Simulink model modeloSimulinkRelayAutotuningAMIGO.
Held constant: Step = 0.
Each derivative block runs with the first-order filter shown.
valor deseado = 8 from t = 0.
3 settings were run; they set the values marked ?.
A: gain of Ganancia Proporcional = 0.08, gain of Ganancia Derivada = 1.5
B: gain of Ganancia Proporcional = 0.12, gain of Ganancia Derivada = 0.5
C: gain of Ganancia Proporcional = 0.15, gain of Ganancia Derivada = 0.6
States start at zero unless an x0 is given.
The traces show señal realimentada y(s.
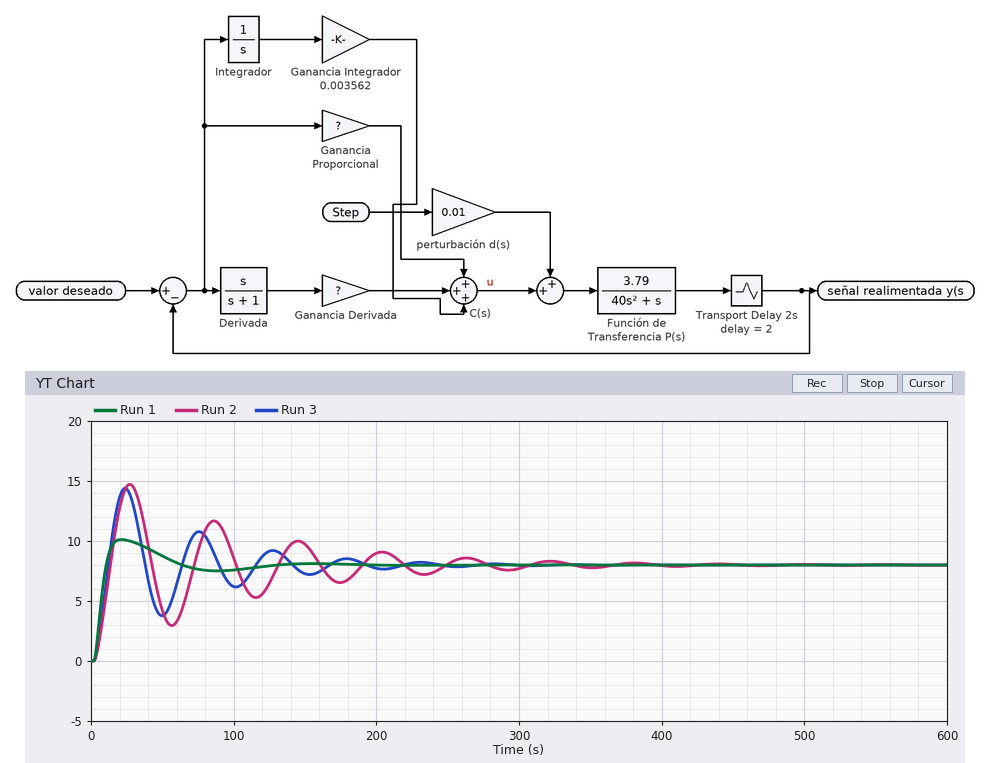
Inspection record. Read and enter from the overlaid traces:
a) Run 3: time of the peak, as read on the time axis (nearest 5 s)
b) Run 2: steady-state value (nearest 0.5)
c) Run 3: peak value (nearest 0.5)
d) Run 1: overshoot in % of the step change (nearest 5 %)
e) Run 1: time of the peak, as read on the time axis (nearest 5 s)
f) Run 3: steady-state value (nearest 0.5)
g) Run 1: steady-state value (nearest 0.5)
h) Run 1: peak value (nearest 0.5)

25 s
8.0
14.5
25 %
20 s
8.0
8.0
10.0
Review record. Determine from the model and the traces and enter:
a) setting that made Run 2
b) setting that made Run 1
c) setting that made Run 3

B
A
C
